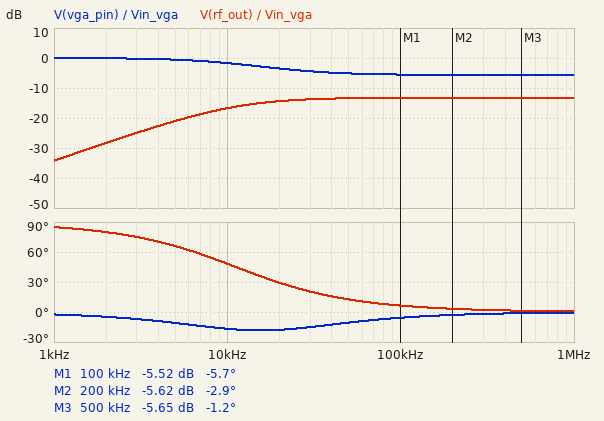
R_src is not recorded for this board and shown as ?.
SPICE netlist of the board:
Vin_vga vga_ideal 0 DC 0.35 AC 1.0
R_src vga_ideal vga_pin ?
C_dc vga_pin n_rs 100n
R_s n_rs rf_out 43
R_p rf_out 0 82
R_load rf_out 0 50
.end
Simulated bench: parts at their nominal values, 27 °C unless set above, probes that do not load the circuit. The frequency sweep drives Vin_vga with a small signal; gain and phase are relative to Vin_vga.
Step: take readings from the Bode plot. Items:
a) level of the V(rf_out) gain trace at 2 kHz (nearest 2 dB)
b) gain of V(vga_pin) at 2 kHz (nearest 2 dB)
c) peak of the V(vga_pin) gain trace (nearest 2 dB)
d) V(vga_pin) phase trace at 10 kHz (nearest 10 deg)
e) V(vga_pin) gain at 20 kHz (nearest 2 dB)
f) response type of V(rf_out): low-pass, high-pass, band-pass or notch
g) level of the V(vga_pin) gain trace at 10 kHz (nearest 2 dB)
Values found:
-28 dB
0 dB
0 dB
-20 deg
-4 dB
high-pass
-2 dB
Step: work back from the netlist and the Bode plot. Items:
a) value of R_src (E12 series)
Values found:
68 Ω
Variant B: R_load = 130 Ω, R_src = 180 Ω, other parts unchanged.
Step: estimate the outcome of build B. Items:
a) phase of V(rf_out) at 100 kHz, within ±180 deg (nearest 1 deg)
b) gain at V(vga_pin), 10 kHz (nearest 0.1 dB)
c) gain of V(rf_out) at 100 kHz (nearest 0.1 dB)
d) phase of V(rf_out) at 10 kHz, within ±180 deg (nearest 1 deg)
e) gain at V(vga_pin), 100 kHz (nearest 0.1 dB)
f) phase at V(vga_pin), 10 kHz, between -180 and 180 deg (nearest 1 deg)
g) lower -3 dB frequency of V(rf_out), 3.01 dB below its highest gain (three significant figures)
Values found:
3 deg
-4.7 dB
-14.7 dB
30 deg
-9.2 dB
-29 deg
5.82 kHz
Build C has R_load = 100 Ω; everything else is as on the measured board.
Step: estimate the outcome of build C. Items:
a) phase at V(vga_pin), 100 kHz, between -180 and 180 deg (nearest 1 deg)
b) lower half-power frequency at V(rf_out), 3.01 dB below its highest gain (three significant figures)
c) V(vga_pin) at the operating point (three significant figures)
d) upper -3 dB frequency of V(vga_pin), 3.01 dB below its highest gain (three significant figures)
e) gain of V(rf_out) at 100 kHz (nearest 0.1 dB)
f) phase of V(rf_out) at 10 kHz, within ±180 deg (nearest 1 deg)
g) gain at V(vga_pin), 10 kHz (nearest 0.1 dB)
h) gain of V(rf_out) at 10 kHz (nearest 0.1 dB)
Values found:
-4 deg
10.2 kHz
350 mV
16.9 kHz
-10.8 dB
46 deg
-1.8 dB
-13.9 dB
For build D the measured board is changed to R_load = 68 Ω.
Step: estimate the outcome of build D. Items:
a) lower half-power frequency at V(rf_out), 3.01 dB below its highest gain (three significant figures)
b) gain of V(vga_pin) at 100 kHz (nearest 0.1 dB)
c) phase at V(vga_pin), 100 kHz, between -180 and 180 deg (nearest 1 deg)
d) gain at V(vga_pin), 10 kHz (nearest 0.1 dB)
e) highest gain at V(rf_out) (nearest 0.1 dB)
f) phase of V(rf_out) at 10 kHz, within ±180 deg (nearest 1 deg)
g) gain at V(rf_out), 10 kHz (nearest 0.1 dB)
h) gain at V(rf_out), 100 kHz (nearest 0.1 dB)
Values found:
10.7 kHz
-5.2 dB
-5 deg
-1.7 dB
-12.0 dB
47 deg
-15.3 dB
-12.1 dB
